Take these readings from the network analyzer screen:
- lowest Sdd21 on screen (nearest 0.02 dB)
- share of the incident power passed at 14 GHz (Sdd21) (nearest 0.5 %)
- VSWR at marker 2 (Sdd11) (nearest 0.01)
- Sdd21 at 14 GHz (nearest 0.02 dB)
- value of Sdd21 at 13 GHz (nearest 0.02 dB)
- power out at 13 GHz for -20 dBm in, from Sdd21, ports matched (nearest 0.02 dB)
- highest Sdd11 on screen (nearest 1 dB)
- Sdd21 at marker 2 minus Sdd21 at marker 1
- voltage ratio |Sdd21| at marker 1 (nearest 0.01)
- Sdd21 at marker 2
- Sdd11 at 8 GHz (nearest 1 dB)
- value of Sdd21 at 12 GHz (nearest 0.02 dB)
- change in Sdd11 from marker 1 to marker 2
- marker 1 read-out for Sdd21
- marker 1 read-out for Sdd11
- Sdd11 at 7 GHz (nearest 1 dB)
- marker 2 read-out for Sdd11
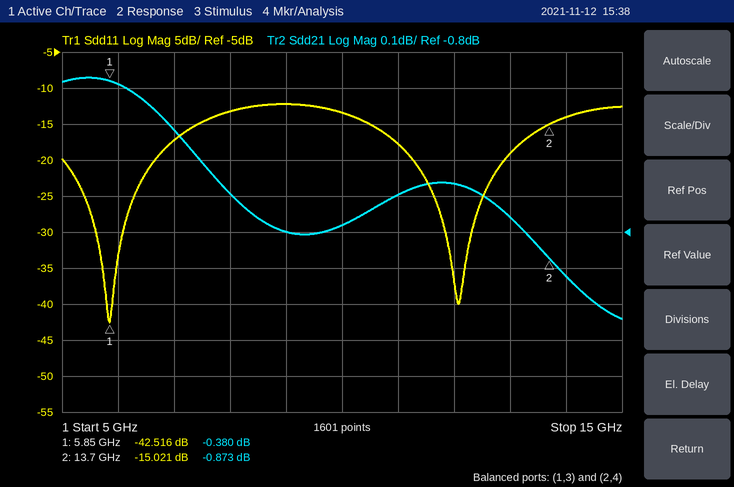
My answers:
-1.04 dB
81.0 %
1.43
-0.92 dB
-0.76 dB
-20.76 dBm
-12 dB
-0.493 dB
0.96
-0.873 dB
-13 dB
-0.66 dB
27.495 dB
-0.380 dB
-42.516 dB
-17 dB
-15.021 dB
